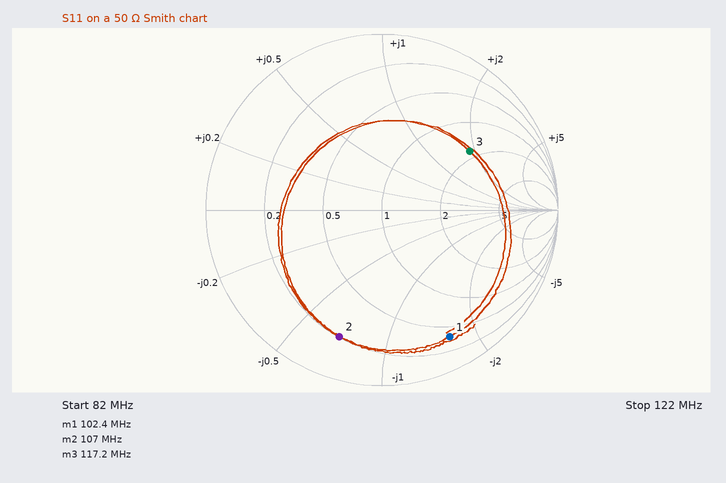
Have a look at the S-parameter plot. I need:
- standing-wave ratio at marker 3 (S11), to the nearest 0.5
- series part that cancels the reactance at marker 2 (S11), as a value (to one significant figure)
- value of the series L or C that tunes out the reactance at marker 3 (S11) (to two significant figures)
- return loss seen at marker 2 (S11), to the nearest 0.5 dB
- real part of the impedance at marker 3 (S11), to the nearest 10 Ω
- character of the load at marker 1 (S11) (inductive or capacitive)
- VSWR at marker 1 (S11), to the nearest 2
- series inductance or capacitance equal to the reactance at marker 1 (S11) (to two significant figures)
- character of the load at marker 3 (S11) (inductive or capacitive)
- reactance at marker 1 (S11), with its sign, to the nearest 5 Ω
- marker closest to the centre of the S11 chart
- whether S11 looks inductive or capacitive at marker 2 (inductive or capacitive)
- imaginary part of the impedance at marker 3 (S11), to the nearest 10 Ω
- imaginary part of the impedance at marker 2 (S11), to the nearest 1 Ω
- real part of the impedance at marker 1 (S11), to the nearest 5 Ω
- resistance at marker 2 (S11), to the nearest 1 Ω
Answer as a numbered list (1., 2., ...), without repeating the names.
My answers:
1. 4.0
2. 50 nH
3. 15 pF
4. 2.5 dB
5. 90 Ω
6. capacitive
7. 10
8. 19 pF
9. inductive
10. -80 Ω
11. marker 3
12. capacitive
13. +90 Ω
14. -35 Ω
15. 20 Ω
16. 10 Ω
